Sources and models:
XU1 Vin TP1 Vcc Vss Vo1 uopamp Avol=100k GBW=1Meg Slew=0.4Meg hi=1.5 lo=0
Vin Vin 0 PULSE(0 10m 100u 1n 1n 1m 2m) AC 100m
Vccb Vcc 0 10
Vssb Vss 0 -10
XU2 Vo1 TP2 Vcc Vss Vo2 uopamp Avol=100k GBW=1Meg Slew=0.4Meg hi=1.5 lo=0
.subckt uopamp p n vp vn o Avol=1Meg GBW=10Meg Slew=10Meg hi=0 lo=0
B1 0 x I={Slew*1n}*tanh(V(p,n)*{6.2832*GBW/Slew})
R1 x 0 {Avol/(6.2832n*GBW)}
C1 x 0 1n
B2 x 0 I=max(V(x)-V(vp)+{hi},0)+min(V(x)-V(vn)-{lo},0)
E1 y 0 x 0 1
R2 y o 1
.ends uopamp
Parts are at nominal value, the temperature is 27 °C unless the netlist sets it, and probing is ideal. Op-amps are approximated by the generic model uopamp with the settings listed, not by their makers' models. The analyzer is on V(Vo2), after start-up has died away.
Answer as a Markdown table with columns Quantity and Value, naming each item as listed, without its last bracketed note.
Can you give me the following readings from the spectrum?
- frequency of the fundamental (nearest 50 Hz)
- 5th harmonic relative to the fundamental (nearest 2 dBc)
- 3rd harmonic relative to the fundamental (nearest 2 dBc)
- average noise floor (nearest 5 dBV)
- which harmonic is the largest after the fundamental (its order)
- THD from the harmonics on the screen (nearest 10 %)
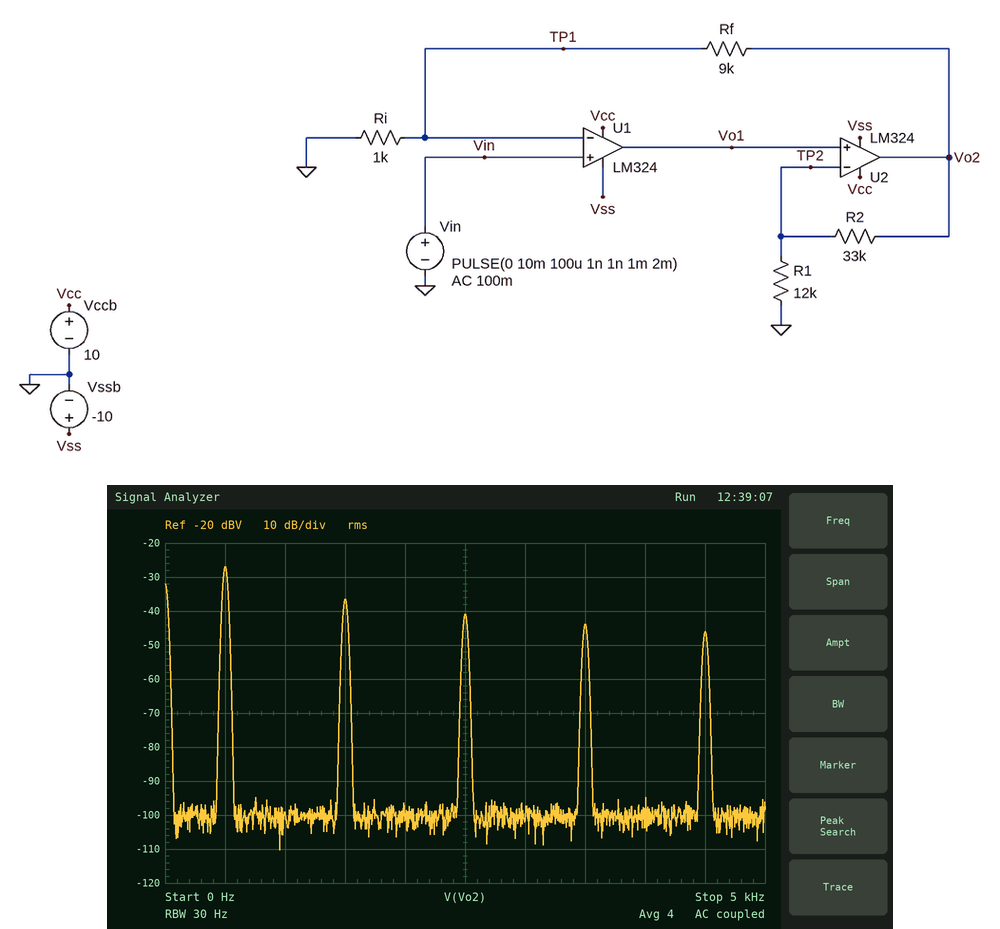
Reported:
| Quantity | Value |
|---|---|
| frequency of the fundamental | 500 Hz |
| 5th harmonic relative to the fundamental | -14 dBc |
| 3rd harmonic relative to the fundamental | -10 dBc |
| average noise floor | -100 dBV |
| which harmonic is the largest after the fundamental | 3 |
| THD from the harmonics on the screen | 40 % |
